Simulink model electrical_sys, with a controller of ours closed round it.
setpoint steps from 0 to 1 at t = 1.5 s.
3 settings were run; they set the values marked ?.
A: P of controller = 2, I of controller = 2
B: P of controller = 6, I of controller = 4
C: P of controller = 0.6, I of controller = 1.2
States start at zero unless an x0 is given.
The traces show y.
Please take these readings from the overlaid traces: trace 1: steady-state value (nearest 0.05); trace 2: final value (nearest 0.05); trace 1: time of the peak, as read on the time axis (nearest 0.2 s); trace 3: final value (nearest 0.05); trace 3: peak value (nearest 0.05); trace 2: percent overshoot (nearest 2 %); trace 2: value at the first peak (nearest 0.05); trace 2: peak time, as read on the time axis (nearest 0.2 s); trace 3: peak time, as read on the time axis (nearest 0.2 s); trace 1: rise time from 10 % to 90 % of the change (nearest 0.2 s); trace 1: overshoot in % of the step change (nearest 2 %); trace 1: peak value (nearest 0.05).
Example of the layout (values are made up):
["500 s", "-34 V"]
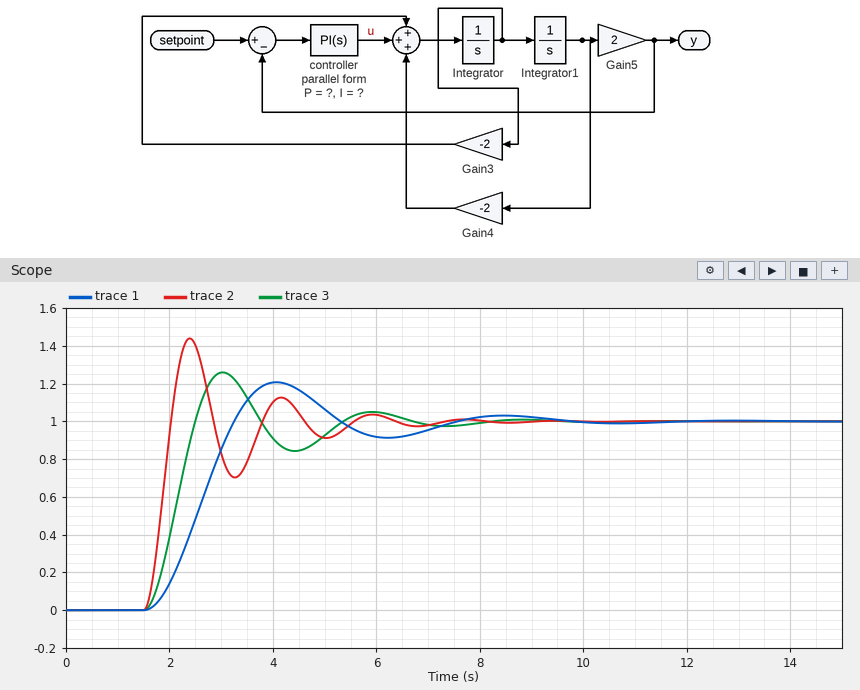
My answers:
["1.00", "1.00", "4.0 s", "1.00", "1.25", "44 %", "1.45", "2.4 s", "3.0 s", "1.2 s", "20 %", "1.20"]
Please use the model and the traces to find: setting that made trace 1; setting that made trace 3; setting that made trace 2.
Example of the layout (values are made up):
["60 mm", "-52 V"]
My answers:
["C", "A", "B"]
